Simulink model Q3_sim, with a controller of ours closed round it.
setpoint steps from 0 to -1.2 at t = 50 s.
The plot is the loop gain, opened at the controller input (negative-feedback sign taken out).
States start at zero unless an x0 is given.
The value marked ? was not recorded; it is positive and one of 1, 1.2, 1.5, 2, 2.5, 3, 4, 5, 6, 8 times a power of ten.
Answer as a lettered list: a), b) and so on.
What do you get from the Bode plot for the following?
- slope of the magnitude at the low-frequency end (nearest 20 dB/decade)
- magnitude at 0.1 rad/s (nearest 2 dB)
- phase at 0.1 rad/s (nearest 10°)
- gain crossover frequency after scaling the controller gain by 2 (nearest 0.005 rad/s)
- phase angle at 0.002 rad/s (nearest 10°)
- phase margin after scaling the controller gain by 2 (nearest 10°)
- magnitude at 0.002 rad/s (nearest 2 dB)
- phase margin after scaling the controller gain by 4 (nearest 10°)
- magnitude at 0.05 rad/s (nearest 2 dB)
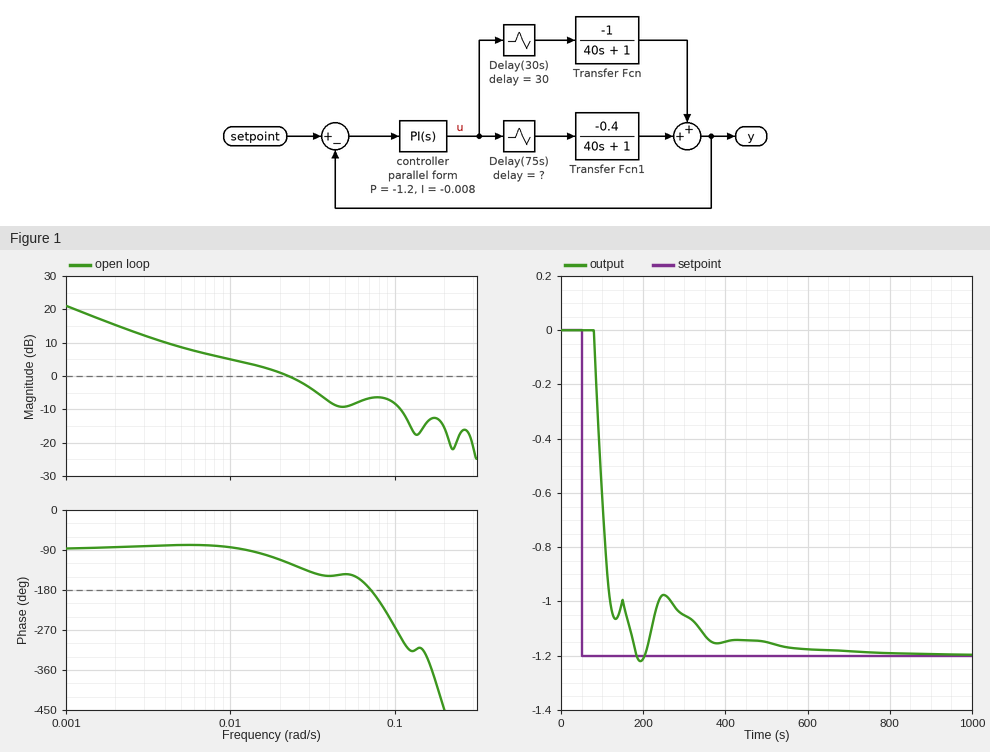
a) -20 dB/decade
b) -8 dB
c) -260°
d) 0.035 rad/s
e) -80°
f) 30°
g) 16 dB
h) -120°
i) -10 dB
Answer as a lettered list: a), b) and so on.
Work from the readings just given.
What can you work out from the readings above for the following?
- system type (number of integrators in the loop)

a) 1
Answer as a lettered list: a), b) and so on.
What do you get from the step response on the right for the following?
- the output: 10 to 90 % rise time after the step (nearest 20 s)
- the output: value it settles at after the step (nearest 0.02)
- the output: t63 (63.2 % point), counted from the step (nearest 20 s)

a) 80 s
b) -1.20
c) 60 s
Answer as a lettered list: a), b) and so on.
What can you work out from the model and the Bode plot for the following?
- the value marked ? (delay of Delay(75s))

a) 100
